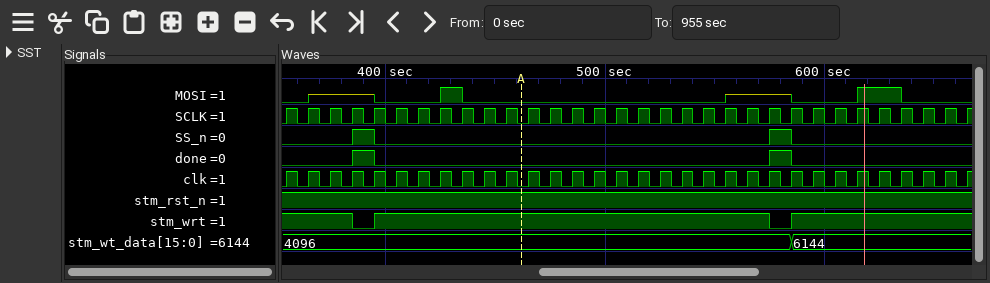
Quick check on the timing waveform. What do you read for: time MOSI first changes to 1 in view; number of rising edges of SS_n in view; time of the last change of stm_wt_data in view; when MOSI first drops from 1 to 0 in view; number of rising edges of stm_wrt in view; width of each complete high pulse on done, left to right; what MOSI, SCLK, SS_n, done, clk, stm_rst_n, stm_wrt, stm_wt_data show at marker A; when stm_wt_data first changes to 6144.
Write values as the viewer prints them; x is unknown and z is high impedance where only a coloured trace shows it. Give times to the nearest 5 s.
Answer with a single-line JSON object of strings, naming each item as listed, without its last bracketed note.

{"time MOSI first changes to 1 in view": "425 s", "number of rising edges of SS_n in view": "2", "time of the last change of stm_wt_data in view": "585 s", "when MOSI first drops from 1 to 0 in view": "435 s", "number of rising edges of stm_wrt in view": "2", "width of each complete high pulse on done, left to right": "10 s, 10 s", "what MOSI, SCLK, SS_n, done, clk, stm_rst_n, stm_wrt, stm_wt_data show at marker A": "MOSI=0, SCLK=0, SS_n=0, done=0, clk=0, stm_rst_n=1, stm_wrt=1, stm_wt_data=4096", "when stm_wt_data first changes to 6144": "585 s"}
